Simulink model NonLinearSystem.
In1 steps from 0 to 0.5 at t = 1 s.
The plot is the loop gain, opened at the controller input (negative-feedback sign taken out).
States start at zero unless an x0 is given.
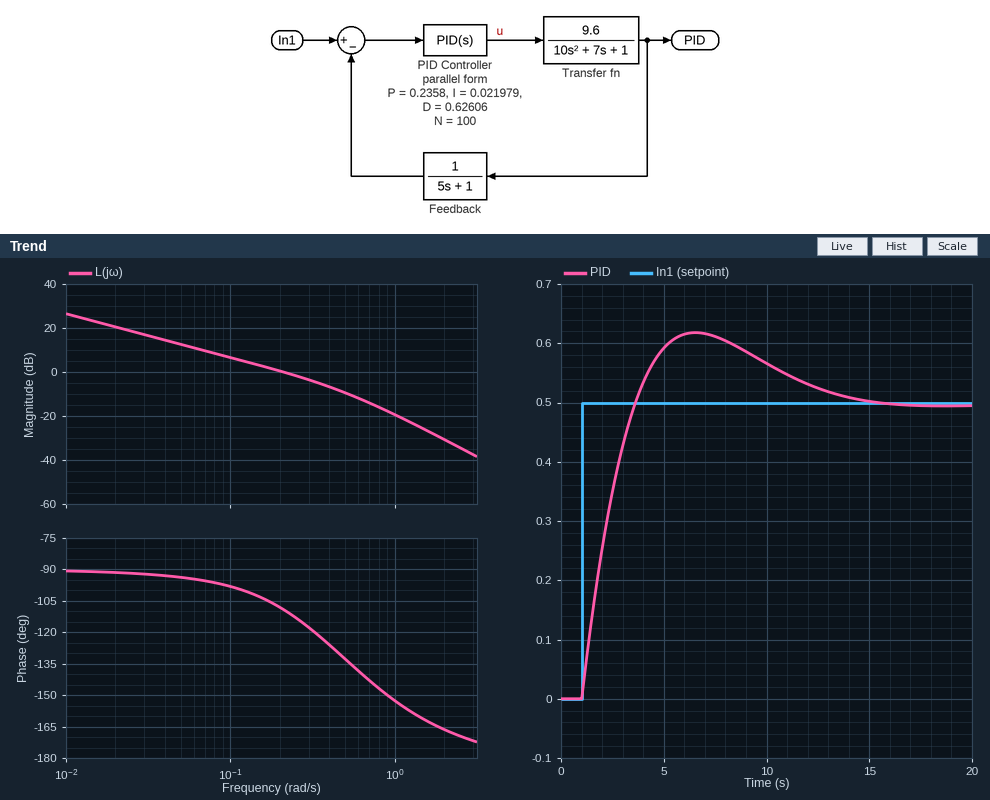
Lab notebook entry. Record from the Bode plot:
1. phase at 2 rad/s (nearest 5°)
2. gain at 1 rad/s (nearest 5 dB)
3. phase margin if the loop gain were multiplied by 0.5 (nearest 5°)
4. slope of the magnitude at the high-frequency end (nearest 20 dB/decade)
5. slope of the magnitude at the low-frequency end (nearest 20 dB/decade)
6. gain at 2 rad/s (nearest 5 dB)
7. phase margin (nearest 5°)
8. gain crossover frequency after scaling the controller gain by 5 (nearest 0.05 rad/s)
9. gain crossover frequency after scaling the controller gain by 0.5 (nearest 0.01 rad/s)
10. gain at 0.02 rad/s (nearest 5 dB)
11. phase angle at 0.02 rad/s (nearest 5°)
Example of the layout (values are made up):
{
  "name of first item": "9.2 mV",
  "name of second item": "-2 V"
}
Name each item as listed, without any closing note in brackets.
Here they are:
{
  "phase at 2 rad/s": "-165°",
  "gain at 1 rad/s": "-20 dB",
  "phase margin if the loop gain were multiplied by 0.5": "80°",
  "slope of the magnitude at the high-frequency end": "-40 dB/decade",
  "slope of the magnitude at the low-frequency end": "-20 dB/decade",
  "gain at 2 rad/s": "-30 dB",
  "phase margin": "70°",
  "gain crossover frequency after scaling the controller gain by 5": "0.70 rad/s",
  "gain crossover frequency after scaling the controller gain by 0.5": "0.11 rad/s",
  "gain at 0.02 rad/s": "20 dB",
  "phase angle at 0.02 rad/s": "-90°"
}
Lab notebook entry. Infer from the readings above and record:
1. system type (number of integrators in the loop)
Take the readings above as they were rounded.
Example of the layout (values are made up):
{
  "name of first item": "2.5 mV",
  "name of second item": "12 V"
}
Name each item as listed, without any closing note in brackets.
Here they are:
{
  "system type": "1"
}
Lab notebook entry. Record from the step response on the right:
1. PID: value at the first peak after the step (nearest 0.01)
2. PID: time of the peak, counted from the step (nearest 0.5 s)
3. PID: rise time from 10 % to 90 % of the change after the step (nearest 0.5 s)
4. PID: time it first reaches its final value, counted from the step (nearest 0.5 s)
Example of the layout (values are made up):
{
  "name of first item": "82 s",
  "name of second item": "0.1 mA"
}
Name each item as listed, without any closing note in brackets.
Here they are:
{
  "PID: value at the first peak after the step": "0.62",
  "PID: time of the peak, counted from the step": "5.5 s",
  "PID: rise time from 10 % to 90 % of the change after the step": "2.0 s",
  "PID: time it first reaches its final value, counted from the step": "2.5 s"
}
